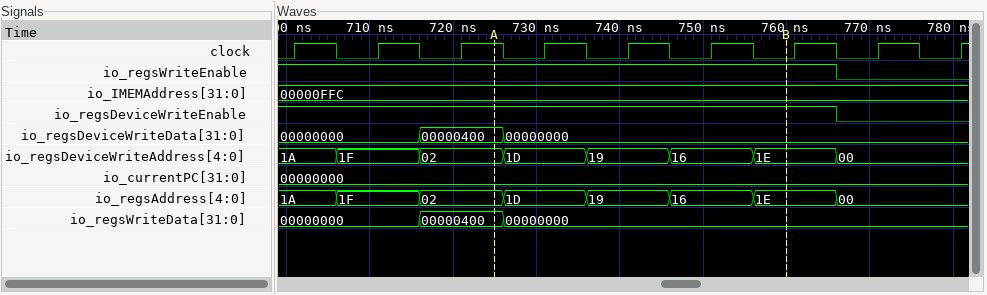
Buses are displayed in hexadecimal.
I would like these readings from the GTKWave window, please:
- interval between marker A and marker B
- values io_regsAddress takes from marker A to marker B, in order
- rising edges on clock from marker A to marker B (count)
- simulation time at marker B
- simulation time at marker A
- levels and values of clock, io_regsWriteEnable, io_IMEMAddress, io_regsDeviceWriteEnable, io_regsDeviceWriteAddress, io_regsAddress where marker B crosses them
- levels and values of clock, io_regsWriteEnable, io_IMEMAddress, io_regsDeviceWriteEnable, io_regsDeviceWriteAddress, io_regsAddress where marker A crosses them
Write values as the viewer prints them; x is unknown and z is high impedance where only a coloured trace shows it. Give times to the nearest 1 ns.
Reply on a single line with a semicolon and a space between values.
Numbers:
35 ns; 02, 1D, 19, 16, 1E; 3; 760 ns; 725 ns; clock=0, io_regsWriteEnable=1, io_IMEMAddress=00000FFC, io_regsDeviceWriteEnable=1, io_regsDeviceWriteAddress=1E, io_regsAddress=1E; clock=1, io_regsWriteEnable=1, io_IMEMAddress=00000FFC, io_regsDeviceWriteEnable=1, io_regsDeviceWriteAddress=02, io_regsAddress=02
